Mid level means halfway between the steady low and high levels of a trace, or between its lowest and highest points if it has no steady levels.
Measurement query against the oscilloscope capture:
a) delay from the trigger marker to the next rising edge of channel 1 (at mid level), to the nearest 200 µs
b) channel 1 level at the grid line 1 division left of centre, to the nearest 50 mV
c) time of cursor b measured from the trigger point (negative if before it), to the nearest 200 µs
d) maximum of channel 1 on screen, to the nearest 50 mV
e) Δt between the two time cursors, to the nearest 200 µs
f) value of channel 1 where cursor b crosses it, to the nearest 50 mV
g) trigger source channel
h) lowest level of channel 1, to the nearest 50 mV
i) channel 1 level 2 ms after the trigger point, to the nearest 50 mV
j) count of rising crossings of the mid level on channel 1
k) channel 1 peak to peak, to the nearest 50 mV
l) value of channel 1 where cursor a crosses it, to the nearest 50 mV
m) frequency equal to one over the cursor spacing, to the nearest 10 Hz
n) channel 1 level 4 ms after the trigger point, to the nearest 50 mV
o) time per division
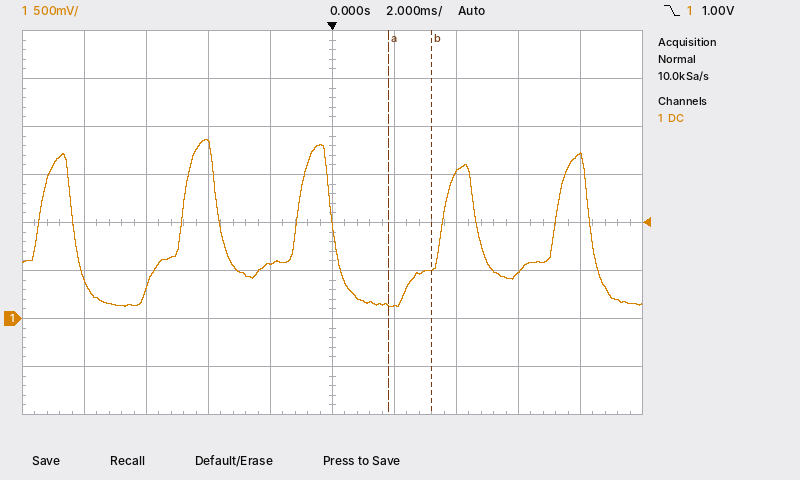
3.6 ms
550 mV
+3.2 ms
1.85 V
1.4 ms
500 mV
channel 1
100 mV
150 mV
5
1.75 V
150 mV
710 Hz
1.50 V
2 ms
